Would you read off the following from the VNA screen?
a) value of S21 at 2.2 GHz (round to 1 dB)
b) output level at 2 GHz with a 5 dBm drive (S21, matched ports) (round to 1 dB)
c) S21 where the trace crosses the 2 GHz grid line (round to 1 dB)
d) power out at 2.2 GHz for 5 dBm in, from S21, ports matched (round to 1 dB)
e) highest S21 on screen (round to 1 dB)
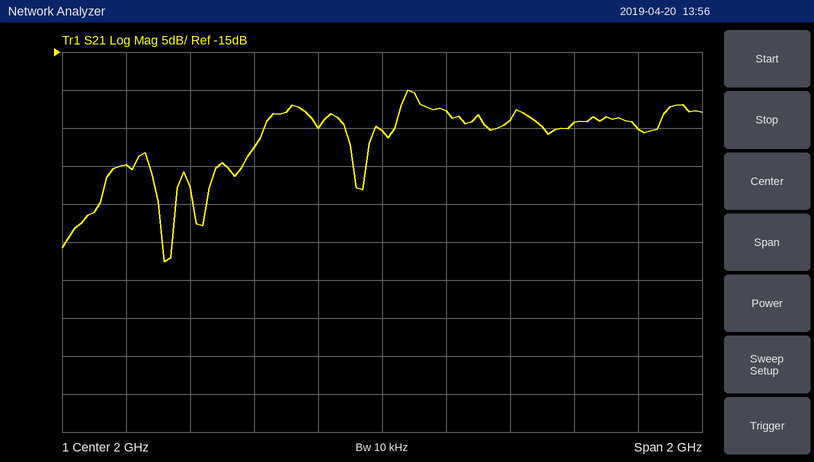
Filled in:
-23 dB
-20 dBm
-25 dB
-18 dBm
-20 dB
